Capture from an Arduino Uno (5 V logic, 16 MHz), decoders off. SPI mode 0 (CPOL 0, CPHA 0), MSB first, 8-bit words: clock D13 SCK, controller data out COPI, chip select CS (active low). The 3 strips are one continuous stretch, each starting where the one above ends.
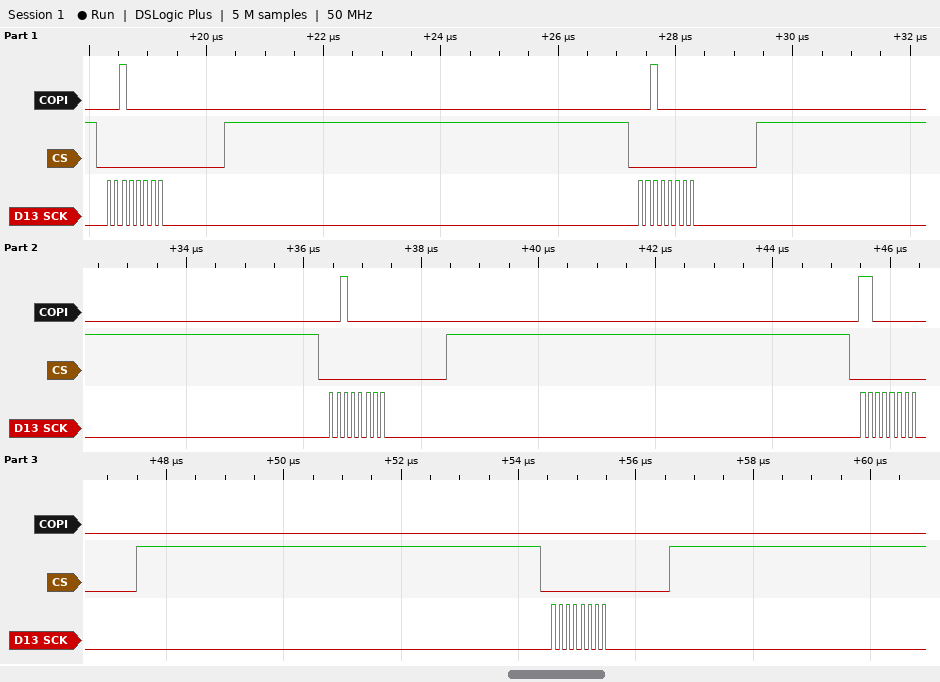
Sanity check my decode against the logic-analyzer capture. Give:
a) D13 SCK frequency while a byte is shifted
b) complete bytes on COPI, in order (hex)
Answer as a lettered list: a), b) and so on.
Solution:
a) 8 MHz
b) 20 20 20 C0 00
